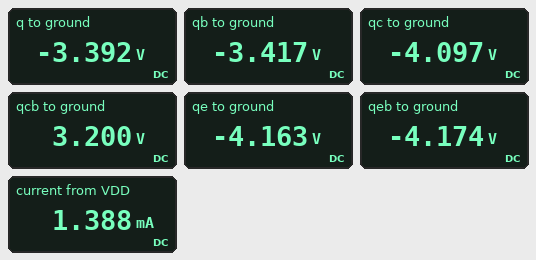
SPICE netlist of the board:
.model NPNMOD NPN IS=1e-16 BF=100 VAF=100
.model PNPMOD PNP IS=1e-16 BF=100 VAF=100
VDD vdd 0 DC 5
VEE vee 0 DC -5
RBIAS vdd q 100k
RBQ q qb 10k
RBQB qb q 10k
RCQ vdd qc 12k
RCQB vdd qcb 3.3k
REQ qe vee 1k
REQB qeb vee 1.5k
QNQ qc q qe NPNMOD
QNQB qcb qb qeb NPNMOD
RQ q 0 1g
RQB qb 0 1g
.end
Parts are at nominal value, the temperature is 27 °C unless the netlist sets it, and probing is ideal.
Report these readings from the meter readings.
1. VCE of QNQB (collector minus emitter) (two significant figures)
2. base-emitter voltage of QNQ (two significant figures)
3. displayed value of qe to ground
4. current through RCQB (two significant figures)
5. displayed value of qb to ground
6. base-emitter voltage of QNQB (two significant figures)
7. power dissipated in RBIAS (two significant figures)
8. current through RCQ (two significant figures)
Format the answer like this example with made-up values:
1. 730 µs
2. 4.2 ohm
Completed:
1. 7.4 V
2. 770 mV
3. -4.163 V
4. 550 µA
5. -3.417 V
6. 760 mV
7. 700 µW
8. 760 µA
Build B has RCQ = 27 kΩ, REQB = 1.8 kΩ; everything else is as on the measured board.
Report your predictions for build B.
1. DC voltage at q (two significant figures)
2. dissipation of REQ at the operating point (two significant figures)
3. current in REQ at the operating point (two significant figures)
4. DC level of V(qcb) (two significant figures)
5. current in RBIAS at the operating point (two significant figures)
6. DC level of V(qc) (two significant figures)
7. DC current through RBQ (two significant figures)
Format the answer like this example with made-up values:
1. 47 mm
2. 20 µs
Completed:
1. -3.8 V
2. 190 µW
3. 440 µA
4. 4.2 V
5. 88 µA
6. -4.5 V
7. 1.1 µA
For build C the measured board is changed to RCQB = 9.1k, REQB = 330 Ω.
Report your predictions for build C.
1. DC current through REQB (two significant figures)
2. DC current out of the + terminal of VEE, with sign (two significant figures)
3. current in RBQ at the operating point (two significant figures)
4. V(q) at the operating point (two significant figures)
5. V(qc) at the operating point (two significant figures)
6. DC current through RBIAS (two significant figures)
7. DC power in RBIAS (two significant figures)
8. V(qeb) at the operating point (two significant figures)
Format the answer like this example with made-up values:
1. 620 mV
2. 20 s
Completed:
1. 1.1 mA
2. -1.9 mA
3. 38 µA
4. -3.5 V
5. -4.1 V
6. 85 µA
7. 720 µW
8. -4.6 V
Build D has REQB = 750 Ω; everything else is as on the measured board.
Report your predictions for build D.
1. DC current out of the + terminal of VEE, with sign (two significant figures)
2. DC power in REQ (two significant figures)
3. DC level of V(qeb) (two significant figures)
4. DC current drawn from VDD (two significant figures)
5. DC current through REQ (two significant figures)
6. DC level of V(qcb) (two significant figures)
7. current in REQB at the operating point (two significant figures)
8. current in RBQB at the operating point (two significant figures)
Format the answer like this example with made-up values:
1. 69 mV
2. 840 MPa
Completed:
1. -1.9 mA
2. 690 µW
3. -4.2 V
4. 1.9 mA
5. 830 µA
6. 1.6 V
7. 1.0 mA
8. 4.9 µA
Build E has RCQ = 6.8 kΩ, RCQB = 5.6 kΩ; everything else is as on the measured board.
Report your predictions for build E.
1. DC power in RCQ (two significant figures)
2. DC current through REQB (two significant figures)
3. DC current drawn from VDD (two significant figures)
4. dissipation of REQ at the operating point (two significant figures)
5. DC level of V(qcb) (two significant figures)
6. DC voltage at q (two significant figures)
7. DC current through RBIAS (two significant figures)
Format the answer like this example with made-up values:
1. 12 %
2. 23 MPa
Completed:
1. 11 mW
2. 870 µA
3. 2.2 mA
4. 1.8 mW
5. 180 mV
6. -2.9 V
7. 79 µA
